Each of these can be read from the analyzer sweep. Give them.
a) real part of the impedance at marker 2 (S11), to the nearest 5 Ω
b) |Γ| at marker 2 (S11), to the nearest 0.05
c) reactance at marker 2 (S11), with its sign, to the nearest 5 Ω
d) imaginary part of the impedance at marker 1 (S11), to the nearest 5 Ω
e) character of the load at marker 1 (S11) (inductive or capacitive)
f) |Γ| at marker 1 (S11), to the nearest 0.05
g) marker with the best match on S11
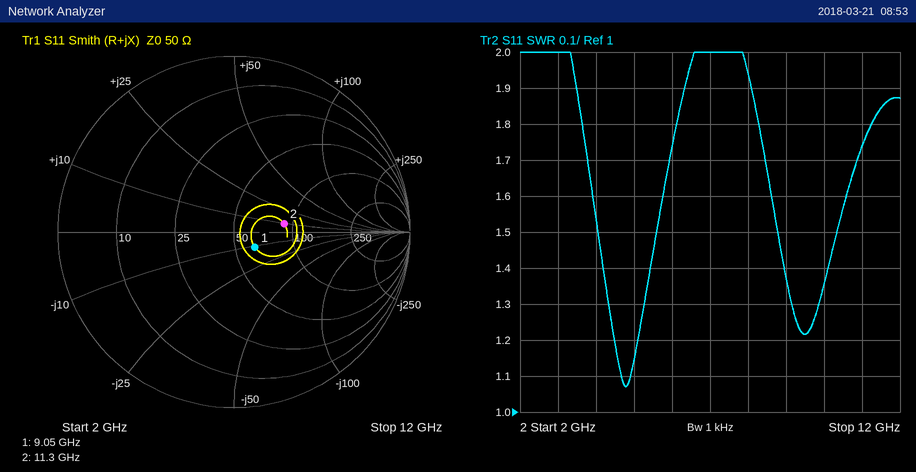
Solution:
90 Ω
0.30
+10 Ω
-10 Ω
capacitive
0.15
marker 1
